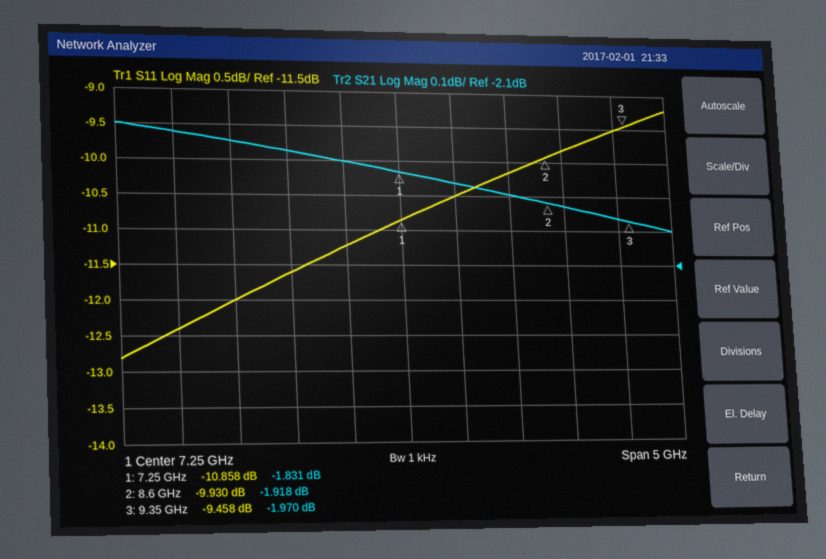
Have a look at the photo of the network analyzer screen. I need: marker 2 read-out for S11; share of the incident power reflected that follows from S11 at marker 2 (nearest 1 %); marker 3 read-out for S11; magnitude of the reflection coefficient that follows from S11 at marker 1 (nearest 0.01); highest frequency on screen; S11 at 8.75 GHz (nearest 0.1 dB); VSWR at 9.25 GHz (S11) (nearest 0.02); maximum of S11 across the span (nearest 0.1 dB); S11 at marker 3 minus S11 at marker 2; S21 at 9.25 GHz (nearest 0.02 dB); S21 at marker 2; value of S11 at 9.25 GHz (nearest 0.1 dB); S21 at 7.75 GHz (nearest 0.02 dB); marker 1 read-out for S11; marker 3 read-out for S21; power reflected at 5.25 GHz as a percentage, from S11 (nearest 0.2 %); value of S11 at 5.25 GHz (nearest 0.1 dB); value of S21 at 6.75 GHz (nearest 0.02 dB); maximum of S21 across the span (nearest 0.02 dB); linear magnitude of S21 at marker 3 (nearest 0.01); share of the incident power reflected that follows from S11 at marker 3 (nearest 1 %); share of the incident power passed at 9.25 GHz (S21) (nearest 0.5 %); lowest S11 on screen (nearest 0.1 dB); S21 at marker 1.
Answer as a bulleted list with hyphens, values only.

- -9.930 dB
- 10 %
- -9.458 dB
- 0.29
- 9.75 GHz
- -9.8 dB
- 2.00
- -9.2 dB
- 0.472 dB
- -1.96 dB
- -1.918 dB
- -9.5 dB
- -1.86 dB
- -10.858 dB
- -1.970 dB
- 5.8 %
- -12.4 dB
- -1.80 dB
- -1.70 dB
- 0.80
- 11 %
- 63.5 %
- -12.8 dB
- -1.831 dB
